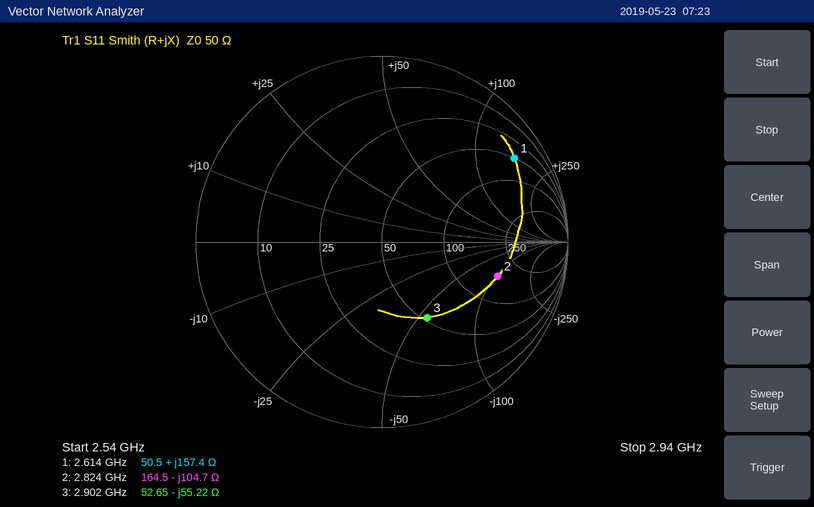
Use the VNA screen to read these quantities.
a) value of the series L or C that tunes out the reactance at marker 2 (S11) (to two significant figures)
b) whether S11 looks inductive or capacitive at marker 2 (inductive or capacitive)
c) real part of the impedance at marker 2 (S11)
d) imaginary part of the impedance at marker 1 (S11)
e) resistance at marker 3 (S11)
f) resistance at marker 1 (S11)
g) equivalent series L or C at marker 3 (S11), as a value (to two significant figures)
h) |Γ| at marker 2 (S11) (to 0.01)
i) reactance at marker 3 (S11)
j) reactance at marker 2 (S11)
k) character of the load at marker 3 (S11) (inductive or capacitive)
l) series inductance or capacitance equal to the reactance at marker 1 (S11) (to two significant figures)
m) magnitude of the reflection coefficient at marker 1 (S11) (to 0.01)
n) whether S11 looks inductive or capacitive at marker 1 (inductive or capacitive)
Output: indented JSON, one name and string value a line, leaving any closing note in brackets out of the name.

{
  "value of the series L or C that tunes out the reactance at marker 2 (S11)": "5.9 nH",
  "whether S11 looks inductive or capacitive at marker 2": "capacitive",
  "real part of the impedance at marker 2": "164.5 Ω",
  "imaginary part of the impedance at marker 1": "+157.4 Ω",
  "resistance at marker 3": "52.65 Ω",
  "resistance at marker 1": "50.5 Ω",
  "equivalent series L or C at marker 3 (S11), as a value": "990 fF",
  "|Γ| at marker 2 (S11)": "0.65",
  "reactance at marker 3": "-55.22 Ω",
  "reactance at marker 2": "-104.7 Ω",
  "character of the load at marker 3 (S11)": "capacitive",
  "series inductance or capacitance equal to the reactance at marker 1 (S11)": "9.6 nH",
  "magnitude of the reflection coefficient at marker 1 (S11)": "0.84",
  "whether S11 looks inductive or capacitive at marker 1": "inductive"
}
